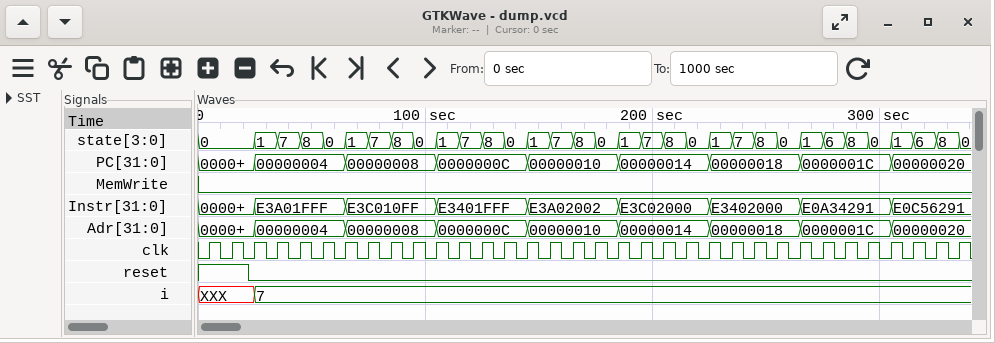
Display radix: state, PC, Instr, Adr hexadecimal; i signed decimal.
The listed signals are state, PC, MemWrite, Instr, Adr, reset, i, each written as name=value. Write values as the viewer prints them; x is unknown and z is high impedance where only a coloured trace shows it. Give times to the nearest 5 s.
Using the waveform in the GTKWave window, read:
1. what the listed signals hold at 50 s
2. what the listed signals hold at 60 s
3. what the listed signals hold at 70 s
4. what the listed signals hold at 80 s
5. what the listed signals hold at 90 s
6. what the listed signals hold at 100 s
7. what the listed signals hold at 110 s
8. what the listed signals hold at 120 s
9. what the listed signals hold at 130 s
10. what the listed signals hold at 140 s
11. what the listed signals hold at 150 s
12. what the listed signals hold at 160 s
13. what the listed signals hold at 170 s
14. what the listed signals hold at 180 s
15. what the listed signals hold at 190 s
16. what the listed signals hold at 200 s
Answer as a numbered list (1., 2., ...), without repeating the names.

1. state=8, PC=00000004, MemWrite=0, Instr=E3A01FFF, Adr=00000004, reset=0, i=7
2. state=0, PC=00000004, MemWrite=0, Instr=E3A01FFF, Adr=00000004, reset=0, i=7
3. state=1, PC=00000008, MemWrite=0, Instr=E3C010FF, Adr=00000008, reset=0, i=7
4. state=7, PC=00000008, MemWrite=0, Instr=E3C010FF, Adr=00000008, reset=0, i=7
5. state=8, PC=00000008, MemWrite=0, Instr=E3C010FF, Adr=00000008, reset=0, i=7
6. state=0, PC=00000008, MemWrite=0, Instr=E3C010FF, Adr=00000008, reset=0, i=7
7. state=1, PC=0000000C, MemWrite=0, Instr=E3401FFF, Adr=0000000C, reset=0, i=7
8. state=7, PC=0000000C, MemWrite=0, Instr=E3401FFF, Adr=0000000C, reset=0, i=7
9. state=8, PC=0000000C, MemWrite=0, Instr=E3401FFF, Adr=0000000C, reset=0, i=7
10. state=0, PC=0000000C, MemWrite=0, Instr=E3401FFF, Adr=0000000C, reset=0, i=7
11. state=1, PC=00000010, MemWrite=0, Instr=E3A02002, Adr=00000010, reset=0, i=7
12. state=7, PC=00000010, MemWrite=0, Instr=E3A02002, Adr=00000010, reset=0, i=7
13. state=8, PC=00000010, MemWrite=0, Instr=E3A02002, Adr=00000010, reset=0, i=7
14. state=0, PC=00000010, MemWrite=0, Instr=E3A02002, Adr=00000010, reset=0, i=7
15. state=1, PC=00000014, MemWrite=0, Instr=E3C02000, Adr=00000014, reset=0, i=7
16. state=7, PC=00000014, MemWrite=0, Instr=E3C02000, Adr=00000014, reset=0, i=7
